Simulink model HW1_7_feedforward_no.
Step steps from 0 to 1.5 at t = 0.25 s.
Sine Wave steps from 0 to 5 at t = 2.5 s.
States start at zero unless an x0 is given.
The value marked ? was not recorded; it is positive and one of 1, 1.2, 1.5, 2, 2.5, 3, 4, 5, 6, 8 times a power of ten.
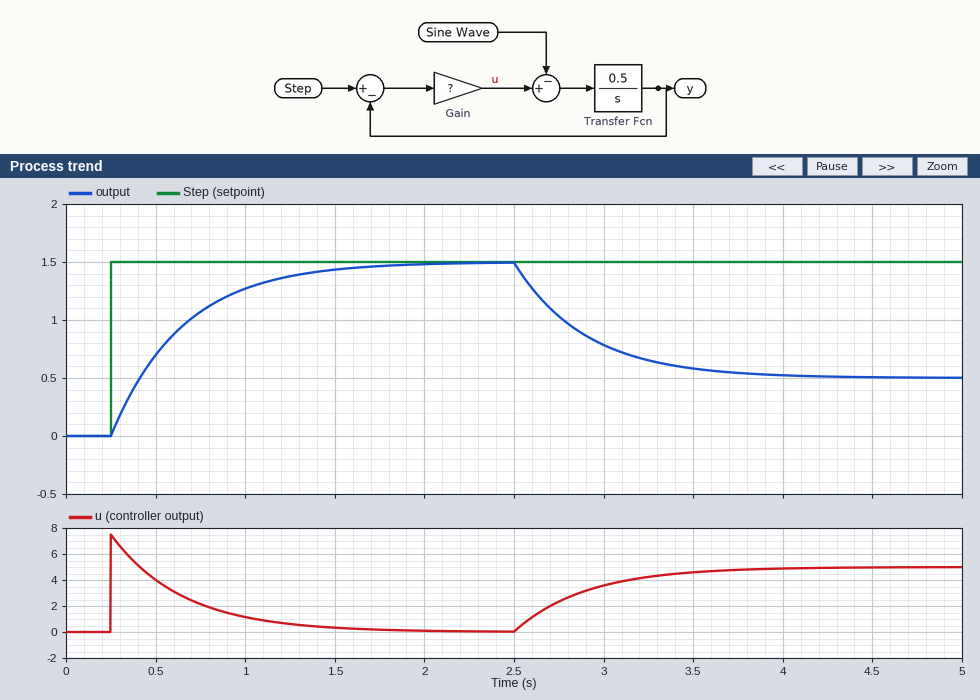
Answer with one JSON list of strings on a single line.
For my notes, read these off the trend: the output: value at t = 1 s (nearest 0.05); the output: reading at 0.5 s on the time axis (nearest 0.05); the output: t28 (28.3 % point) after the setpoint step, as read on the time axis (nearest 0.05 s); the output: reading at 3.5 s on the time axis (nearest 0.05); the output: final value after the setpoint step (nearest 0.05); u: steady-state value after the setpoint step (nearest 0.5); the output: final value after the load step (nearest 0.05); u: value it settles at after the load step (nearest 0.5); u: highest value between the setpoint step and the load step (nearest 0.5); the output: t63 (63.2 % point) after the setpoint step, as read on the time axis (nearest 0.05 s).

["1.25", "0.70", "0.40 s", "0.60", "1.50", "0.0", "0.50", "5.0", "7.5", "0.65 s"]
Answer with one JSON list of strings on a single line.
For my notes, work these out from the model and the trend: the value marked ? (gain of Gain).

["5"]
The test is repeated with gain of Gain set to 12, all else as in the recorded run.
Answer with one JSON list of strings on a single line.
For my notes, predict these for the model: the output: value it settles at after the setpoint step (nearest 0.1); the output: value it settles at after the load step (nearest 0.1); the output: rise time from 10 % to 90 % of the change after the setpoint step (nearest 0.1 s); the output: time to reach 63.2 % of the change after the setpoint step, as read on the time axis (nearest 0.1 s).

["1.5", "1.1", "0.4 s", "0.4 s"]
